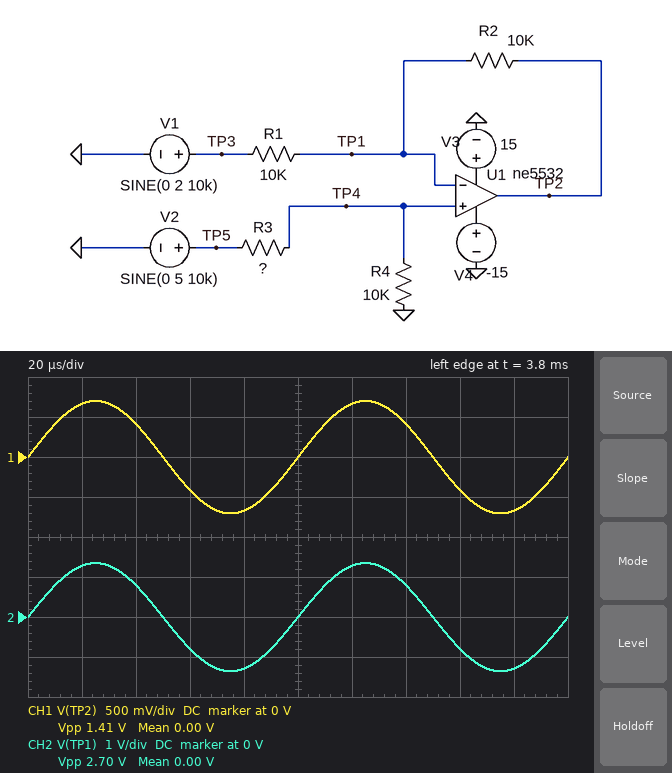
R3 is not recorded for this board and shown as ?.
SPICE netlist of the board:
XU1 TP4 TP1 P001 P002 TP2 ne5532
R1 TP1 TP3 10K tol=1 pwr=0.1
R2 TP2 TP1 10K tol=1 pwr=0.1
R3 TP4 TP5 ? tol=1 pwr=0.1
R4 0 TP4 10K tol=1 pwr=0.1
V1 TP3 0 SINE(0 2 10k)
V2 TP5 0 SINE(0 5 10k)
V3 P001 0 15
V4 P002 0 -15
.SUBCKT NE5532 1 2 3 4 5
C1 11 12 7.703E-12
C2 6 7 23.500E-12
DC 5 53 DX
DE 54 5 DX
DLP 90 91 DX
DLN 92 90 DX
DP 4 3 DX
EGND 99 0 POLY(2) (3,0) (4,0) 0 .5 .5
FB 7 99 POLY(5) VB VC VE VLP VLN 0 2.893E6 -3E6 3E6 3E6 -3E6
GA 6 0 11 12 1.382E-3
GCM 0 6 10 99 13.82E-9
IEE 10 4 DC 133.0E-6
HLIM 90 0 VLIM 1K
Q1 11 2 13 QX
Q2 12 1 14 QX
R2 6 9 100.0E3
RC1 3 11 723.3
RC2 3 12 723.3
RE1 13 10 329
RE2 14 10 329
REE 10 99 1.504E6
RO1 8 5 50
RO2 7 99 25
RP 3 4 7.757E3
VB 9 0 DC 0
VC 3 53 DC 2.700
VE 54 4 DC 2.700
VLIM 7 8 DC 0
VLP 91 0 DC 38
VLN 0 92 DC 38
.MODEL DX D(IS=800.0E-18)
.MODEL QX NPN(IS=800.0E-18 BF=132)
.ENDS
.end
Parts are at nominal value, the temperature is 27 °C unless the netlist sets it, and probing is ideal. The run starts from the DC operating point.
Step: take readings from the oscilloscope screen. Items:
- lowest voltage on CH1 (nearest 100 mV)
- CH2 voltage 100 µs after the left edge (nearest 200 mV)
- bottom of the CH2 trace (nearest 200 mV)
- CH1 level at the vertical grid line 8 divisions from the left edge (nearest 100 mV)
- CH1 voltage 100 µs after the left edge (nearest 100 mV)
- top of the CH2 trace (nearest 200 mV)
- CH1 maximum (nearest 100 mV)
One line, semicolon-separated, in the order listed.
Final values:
-700 mV; 0 V; -1.4 V; -400 mV; 0 V; 1.4 V; 700 mV
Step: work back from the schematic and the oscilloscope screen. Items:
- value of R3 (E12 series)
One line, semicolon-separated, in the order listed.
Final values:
27 kΩ
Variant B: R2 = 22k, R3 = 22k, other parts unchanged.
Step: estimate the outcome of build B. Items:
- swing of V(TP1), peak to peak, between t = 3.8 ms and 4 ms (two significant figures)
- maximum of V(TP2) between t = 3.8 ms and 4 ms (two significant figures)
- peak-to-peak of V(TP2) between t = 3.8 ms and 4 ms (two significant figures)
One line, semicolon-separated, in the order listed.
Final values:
3.1 V; 600 mV; 1.2 V
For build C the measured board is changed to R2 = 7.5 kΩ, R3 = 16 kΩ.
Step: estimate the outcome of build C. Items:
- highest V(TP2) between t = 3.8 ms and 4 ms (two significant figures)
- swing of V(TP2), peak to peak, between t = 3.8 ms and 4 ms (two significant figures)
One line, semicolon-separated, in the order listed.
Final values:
1.9 V; 3.7 V
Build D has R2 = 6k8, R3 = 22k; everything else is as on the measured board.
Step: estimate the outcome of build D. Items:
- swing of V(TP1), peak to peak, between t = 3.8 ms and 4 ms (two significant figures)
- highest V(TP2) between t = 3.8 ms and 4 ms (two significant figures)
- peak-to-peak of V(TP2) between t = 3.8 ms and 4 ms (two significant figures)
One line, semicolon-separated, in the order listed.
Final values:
3.1 V; 1.3 V; 2.5 V
